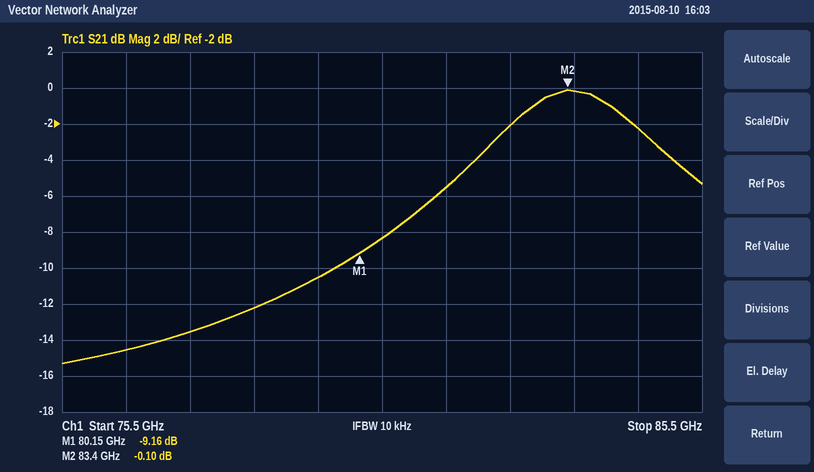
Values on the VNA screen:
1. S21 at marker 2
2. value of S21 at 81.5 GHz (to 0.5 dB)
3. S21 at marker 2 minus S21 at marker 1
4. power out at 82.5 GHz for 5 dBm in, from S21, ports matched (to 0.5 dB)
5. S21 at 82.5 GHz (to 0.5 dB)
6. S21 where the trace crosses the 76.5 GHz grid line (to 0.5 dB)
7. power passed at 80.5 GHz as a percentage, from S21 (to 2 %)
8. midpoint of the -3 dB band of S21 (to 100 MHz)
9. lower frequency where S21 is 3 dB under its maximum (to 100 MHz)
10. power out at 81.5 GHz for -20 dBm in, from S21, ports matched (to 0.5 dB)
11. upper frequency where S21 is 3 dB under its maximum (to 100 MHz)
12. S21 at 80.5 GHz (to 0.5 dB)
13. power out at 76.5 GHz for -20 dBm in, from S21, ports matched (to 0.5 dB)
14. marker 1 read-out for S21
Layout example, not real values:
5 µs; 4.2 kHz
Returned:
-0.10 dB; -5.5 dB; 9.06 dB; 3.0 dBm; -2.0 dB; -14.5 dB; 14 %; 83.5 GHz; 82.2 GHz; -25.5 dBm; 84.8 GHz; -8.5 dB; -34.5 dBm; -9.16 dB
